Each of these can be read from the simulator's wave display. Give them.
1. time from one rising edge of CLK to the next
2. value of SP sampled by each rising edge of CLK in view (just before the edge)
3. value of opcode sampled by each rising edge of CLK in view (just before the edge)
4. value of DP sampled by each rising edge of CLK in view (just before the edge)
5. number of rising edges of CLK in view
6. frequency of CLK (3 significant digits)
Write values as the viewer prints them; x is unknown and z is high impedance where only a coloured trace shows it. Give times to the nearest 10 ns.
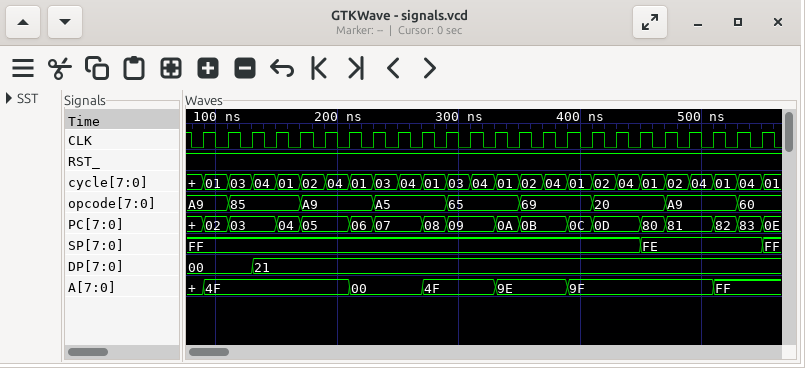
20 ns
FF, FF, FF, FF, FF, FF, FF, FF, FF, FF, FF, FF, FF, FF, FF, FF, FF, FF, FF, FE, FE, FE, FE, FE
A9, A9, 85, 85, 85, A9, A9, A9, A5, A5, A5, 65, 65, 65, 69, 69, 69, 20, 20, 20, A9, A9, A9, 60
00, 00, 00, 21, 21, 21, 21, 21, 21, 21, 21, 21, 21, 21, 21, 21, 21, 21, 21, 21, 21, 21, 21, 21
24
50.0 MHz
